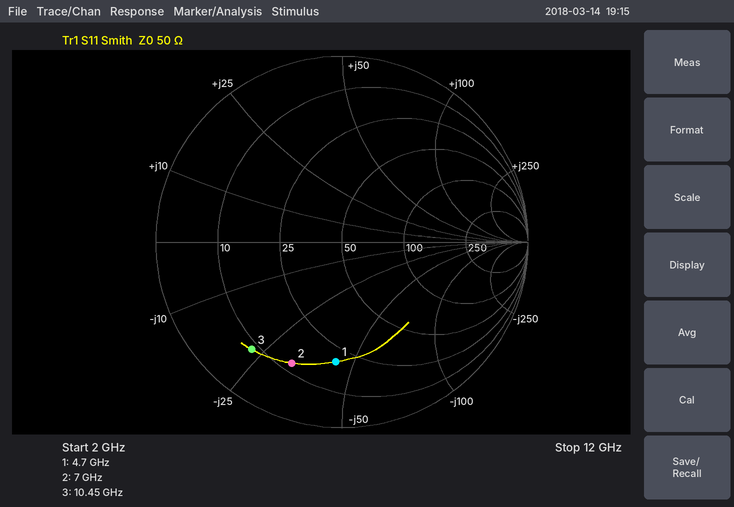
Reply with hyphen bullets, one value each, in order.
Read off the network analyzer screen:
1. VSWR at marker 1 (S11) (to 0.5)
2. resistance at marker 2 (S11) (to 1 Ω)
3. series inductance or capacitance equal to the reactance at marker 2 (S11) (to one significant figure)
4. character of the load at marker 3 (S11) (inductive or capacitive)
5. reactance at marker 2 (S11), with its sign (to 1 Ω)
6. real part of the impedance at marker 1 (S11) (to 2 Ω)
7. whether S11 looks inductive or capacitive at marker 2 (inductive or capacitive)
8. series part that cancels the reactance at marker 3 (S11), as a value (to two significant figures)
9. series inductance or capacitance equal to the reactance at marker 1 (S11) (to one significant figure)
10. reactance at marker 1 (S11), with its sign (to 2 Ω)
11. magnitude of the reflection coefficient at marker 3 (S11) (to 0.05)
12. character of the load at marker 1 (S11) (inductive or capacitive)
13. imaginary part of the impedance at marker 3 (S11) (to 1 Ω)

- 4.5
- 12 Ω
- 700 fF
- capacitive
- -32 Ω
- 20 Ω
- capacitive
- 350 pH
- 800 fF
- -44 Ω
- 0.75
- capacitive
- -23 Ω
